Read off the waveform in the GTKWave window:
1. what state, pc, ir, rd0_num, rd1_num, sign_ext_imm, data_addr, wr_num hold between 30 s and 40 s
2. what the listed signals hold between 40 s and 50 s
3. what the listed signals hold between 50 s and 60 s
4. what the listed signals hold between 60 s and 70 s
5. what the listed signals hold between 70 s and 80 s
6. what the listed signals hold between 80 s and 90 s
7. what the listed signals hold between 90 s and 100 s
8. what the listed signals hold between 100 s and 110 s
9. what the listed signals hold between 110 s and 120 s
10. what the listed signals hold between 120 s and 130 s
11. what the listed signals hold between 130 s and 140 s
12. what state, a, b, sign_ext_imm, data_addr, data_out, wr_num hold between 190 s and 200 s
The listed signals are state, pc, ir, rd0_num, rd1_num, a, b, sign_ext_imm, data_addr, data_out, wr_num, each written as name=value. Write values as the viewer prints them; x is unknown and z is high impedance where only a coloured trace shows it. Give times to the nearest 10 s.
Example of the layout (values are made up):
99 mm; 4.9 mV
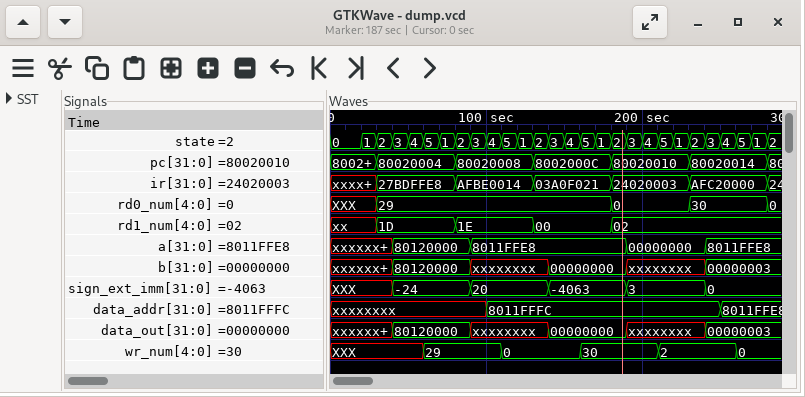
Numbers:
state=2, pc=80020004, ir=27BDFFE8, rd0_num=29, rd1_num=1D, sign_ext_imm=XXX, data_addr=xxxxxxxx, wr_num=XXX; state=3, pc=80020004, ir=27BDFFE8, rd0_num=29, rd1_num=1D, a=80120000, b=80120000, sign_ext_imm=-24, data_addr=xxxxxxxx, data_out=80120000, wr_num=XXX; state=4, pc=80020004, ir=27BDFFE8, rd0_num=29, rd1_num=1D, a=80120000, b=80120000, sign_ext_imm=-24, data_addr=xxxxxxxx, data_out=80120000, wr_num=XXX; state=5, pc=80020004, ir=27BDFFE8, rd0_num=29, rd1_num=1D, a=80120000, b=80120000, sign_ext_imm=-24, data_addr=xxxxxxxx, data_out=80120000, wr_num=29; state=1, pc=80020004, ir=27BDFFE8, rd0_num=29, rd1_num=1D, a=80120000, b=80120000, sign_ext_imm=-24, data_addr=xxxxxxxx, data_out=80120000, wr_num=29; state=2, pc=80020008, ir=AFBE0014, rd0_num=29, rd1_num=1E, a=80120000, b=80120000, sign_ext_imm=-24, data_addr=xxxxxxxx, data_out=80120000, wr_num=29; state=3, pc=80020008, ir=AFBE0014, rd0_num=29, rd1_num=1E, a=8011FFE8, b=xxxxxxxx, sign_ext_imm=20, data_addr=xxxxxxxx, data_out=xxxxxxxx, wr_num=29; state=4, pc=80020008, ir=AFBE0014, rd0_num=29, rd1_num=1E, a=8011FFE8, b=xxxxxxxx, sign_ext_imm=20, data_addr=8011FFFC, data_out=xxxxxxxx, wr_num=29; state=5, pc=80020008, ir=AFBE0014, rd0_num=29, rd1_num=1E, a=8011FFE8, b=xxxxxxxx, sign_ext_imm=20, data_addr=8011FFFC, data_out=xxxxxxxx, wr_num=0; state=1, pc=80020008, ir=AFBE0014, rd0_num=29, rd1_num=1E, a=8011FFE8, b=xxxxxxxx, sign_ext_imm=20, data_addr=8011FFFC, data_out=xxxxxxxx, wr_num=0; state=2, pc=8002000C, ir=03A0F021, rd0_num=29, rd1_num=00, a=8011FFE8, b=xxxxxxxx, sign_ext_imm=20, data_addr=8011FFFC, data_out=xxxxxxxx, wr_num=0; state=3, a=00000000, b=xxxxxxxx, sign_ext_imm=3, data_addr=8011FFFC, data_out=xxxxxxxx, wr_num=30
